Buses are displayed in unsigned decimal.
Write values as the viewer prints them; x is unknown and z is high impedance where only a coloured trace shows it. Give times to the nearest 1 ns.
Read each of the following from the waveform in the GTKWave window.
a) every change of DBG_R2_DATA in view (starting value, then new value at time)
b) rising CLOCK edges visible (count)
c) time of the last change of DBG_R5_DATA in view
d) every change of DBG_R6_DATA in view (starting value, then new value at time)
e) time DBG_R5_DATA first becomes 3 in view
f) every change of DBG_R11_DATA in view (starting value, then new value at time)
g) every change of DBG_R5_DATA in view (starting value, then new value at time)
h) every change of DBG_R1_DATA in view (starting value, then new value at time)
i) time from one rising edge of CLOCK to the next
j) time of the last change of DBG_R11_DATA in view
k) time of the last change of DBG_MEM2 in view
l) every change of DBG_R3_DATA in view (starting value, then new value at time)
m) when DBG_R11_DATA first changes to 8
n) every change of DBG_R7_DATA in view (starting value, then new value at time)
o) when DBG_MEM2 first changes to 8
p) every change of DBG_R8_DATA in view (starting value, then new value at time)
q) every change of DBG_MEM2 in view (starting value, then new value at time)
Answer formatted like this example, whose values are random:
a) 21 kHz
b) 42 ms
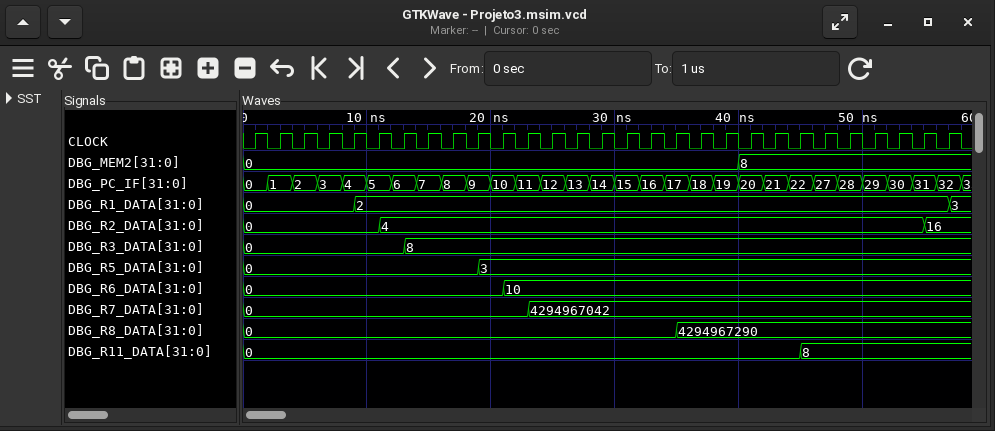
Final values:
a) 0, 4 at 11 ns, 16 at 55 ns
b) 29
c) 19 ns
d) 0, 10 at 21 ns
e) 19 ns
f) 0, 8 at 45 ns
g) 0, 3 at 19 ns
h) 0, 2 at 9 ns, 3 at 57 ns
i) 2 ns
j) 45 ns
k) 40 ns
l) 0, 8 at 13 ns
m) 45 ns
n) 0, 4294967042 at 23 ns
o) 40 ns
p) 0, 4294967290 at 35 ns
q) 0, 8 at 40 ns
